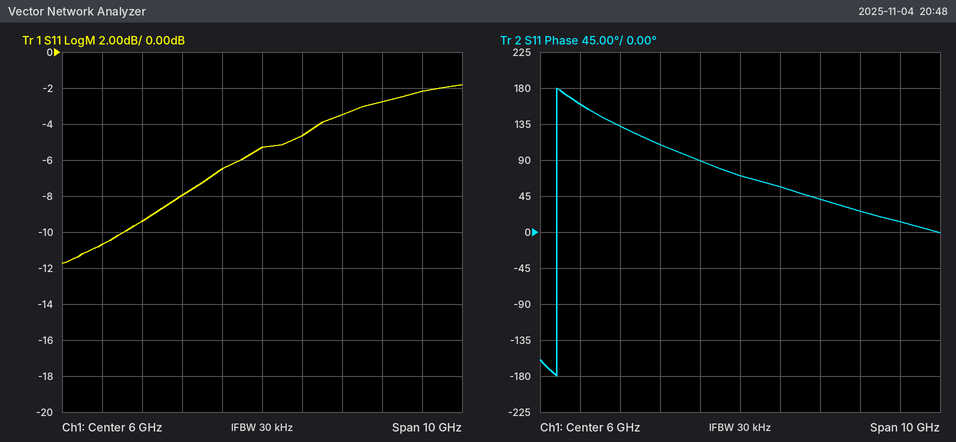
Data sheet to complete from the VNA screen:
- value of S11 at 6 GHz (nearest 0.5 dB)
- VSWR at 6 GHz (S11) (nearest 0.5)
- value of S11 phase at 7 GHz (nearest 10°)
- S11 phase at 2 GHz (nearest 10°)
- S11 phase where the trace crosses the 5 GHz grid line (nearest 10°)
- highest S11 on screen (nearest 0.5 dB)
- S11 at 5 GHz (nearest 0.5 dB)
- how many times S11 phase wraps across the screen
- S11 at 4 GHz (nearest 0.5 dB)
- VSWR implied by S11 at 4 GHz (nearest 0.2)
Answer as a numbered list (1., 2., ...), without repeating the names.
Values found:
1. -5.5 dB
2. 3.5
3. 60°
4. 160°
5. 90°
6. -2.0 dB
7. -6.5 dB
8. 1
9. -8.0 dB
10. 2.4
